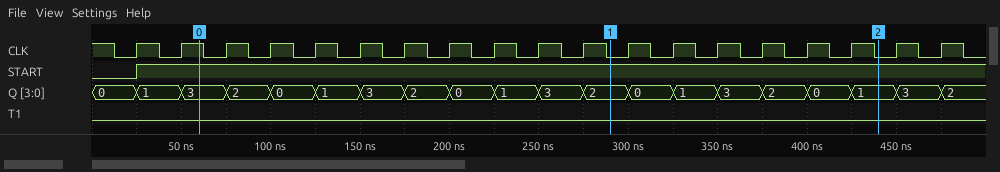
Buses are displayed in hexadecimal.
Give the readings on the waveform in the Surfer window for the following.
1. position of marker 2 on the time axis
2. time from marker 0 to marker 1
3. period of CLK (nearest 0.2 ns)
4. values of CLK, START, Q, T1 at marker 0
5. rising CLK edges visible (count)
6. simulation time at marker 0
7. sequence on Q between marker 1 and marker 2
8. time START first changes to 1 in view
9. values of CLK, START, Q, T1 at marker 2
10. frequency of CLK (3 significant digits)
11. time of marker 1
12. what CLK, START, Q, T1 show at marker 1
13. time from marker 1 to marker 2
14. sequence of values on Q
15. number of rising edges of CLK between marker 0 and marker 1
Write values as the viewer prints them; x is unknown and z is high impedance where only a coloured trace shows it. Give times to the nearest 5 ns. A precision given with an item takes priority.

440 ns
230 ns
25 ns
CLK=1, START=1, Q=3, T1=0
19
60 ns
2, 0, 1, 3, 2, 0, 1
25 ns
CLK=0, START=1, Q=1, T1=0
40.0 MHz
290 ns
CLK=0, START=1, Q=2, T1=0
150 ns
0, 1, 3, 2, 0, 1, 3, 2, 0, 1, 3, 2, 0, 1, 3, 2, 0, 1, 3, 2
9
